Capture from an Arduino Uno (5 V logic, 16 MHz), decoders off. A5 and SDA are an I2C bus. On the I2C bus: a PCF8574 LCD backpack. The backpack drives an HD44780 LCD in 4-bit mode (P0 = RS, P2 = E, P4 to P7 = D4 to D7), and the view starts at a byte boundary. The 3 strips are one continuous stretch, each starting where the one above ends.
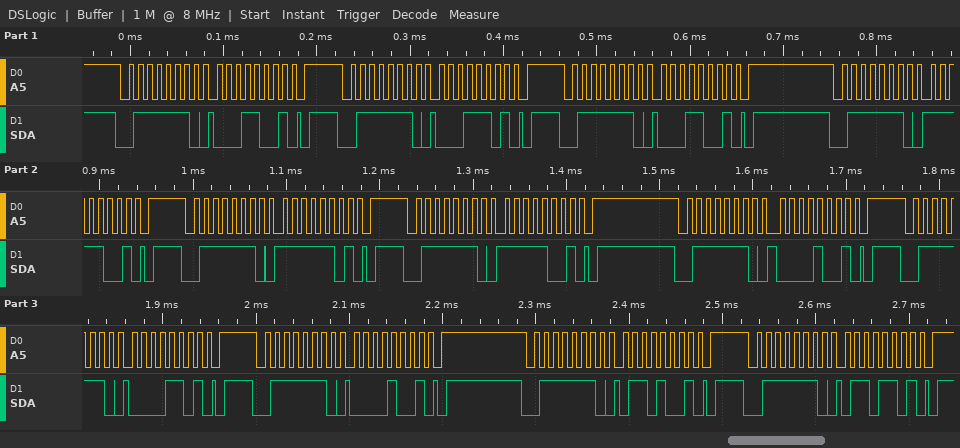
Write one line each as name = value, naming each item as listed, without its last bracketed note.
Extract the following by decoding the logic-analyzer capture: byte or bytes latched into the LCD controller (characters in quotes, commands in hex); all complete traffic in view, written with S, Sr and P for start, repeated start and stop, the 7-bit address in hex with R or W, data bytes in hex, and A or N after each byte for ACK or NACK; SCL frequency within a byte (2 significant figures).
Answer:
byte or bytes latched into the LCD controller = data 0x1F
all complete traffic in view, written with S, Sr and P for start, repeated start and stop, the 7-bit address in hex with R or W, data bytes in hex, and A or N after each byte for ACK or NACK = S 3FW A 19 A P S 3FW A 1D A P S 3FW A 19 A P S 3FW A F9 A P S 3FW A FD A P S 3FW A F9 A P S 3FW A 09 A P S 3FW A 0D A P S 3FW A 09 A P S 3FW A 69 A P S 3FW A 6D A P
SCL frequency within a byte = 100 kHz
